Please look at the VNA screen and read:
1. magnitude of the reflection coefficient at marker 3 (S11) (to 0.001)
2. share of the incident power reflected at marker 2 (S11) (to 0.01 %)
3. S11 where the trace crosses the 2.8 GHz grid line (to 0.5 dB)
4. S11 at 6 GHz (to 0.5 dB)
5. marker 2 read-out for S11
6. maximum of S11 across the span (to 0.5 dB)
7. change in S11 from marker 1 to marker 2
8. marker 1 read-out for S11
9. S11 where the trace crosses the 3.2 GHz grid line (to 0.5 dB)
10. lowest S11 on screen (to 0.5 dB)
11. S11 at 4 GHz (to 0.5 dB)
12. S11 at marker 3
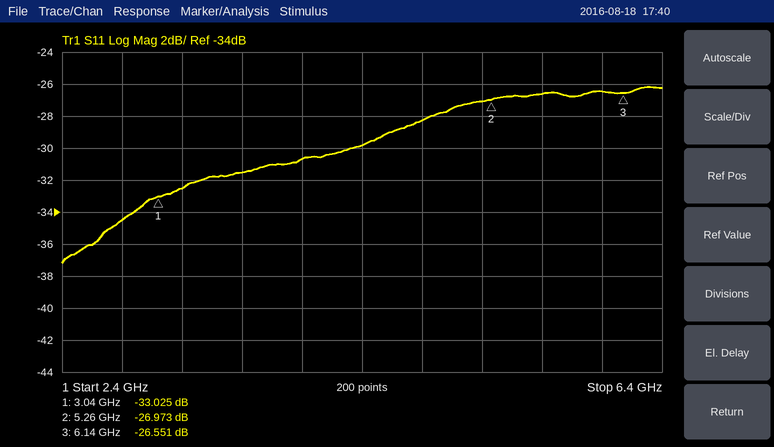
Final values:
0.047
0.20 %
-34.5 dB
-26.5 dB
-26.973 dB
-26.0 dB
6.052 dB
-33.025 dB
-32.5 dB
-37.0 dB
-30.5 dB
-26.551 dB
